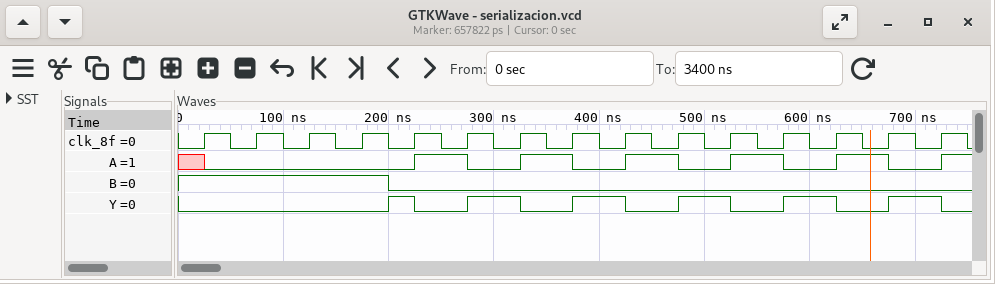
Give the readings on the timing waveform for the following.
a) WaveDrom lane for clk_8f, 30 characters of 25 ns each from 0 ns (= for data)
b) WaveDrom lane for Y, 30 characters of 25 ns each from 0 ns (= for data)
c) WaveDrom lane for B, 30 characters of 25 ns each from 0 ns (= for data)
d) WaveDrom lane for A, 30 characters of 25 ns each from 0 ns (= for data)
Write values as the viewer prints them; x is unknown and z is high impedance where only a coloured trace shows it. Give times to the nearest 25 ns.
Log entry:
{name: 'clk_8f', wave: '010101010101010101010101010101'}
{name: 'Y', wave: '0.......10.1.0.1.0.1.0.1.0.1.0'}
{name: 'B', wave: '1.......0.....................'}
{name: 'A', wave: 'x0.......1.0.1.0.1.0.1.0.1.0.1'}
